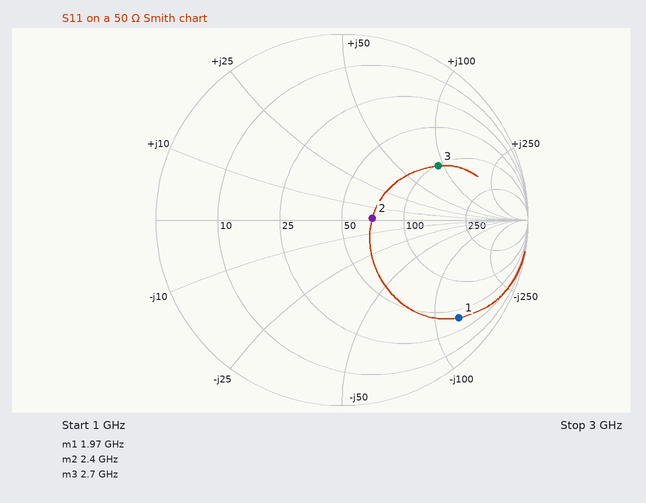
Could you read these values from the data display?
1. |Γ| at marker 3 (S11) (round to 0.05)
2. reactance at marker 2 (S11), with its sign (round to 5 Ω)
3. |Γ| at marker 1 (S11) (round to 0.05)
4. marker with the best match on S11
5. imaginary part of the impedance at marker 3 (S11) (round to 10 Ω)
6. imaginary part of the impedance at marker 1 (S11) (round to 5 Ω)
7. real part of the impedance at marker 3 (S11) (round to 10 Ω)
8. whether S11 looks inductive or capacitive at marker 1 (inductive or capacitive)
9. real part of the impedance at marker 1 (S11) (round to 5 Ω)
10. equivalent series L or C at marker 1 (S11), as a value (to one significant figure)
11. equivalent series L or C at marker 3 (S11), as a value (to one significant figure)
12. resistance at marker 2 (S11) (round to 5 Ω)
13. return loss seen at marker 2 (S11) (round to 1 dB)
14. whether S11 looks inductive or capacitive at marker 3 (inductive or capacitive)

0.60
0 Ω
0.80
marker 2
+90 Ω
-125 Ω
100 Ω
capacitive
40 Ω
600 fF
5 nH
70 Ω
16 dB
inductive
